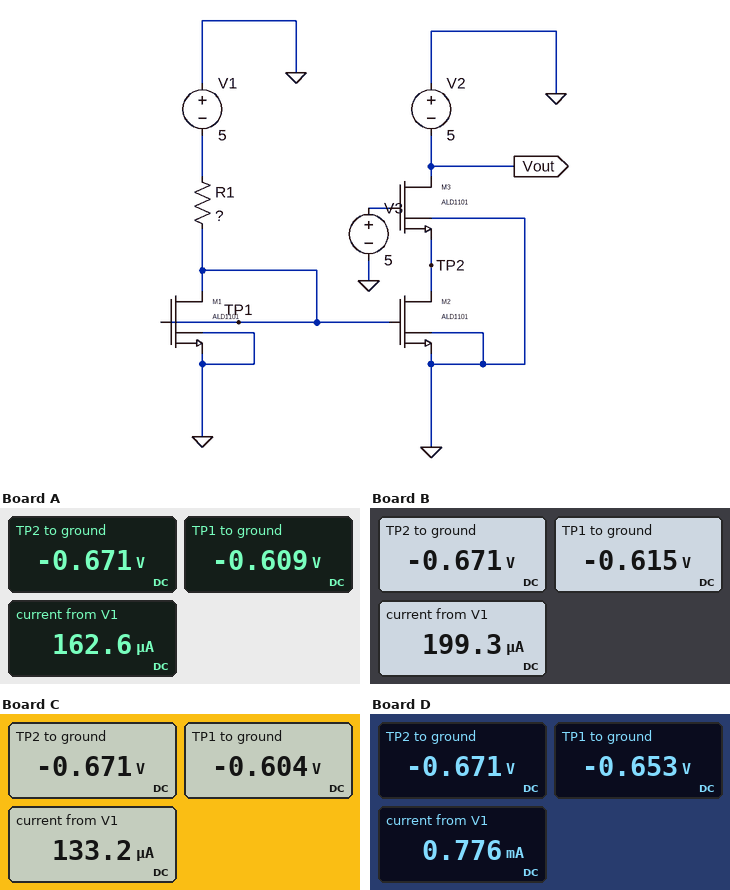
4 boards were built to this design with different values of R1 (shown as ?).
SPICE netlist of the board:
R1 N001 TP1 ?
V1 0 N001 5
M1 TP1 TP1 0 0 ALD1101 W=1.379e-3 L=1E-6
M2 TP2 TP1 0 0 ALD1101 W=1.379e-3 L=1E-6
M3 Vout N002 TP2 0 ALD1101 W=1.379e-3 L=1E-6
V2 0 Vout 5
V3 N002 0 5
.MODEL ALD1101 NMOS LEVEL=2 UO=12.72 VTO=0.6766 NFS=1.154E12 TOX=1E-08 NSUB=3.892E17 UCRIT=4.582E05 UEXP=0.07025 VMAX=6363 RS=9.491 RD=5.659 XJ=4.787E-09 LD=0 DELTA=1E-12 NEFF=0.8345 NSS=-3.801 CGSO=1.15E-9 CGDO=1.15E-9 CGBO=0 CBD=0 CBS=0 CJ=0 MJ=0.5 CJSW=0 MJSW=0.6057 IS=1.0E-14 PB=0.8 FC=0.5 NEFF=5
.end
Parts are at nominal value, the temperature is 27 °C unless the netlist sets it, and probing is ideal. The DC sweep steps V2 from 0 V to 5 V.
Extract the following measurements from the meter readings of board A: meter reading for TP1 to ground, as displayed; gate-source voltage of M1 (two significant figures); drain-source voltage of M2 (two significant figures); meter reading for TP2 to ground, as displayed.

-0.609 V
-610 mV
-670 mV
-0.671 V
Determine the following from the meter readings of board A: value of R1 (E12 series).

27 kΩ
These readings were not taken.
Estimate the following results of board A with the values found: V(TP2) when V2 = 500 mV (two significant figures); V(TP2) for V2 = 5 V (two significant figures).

-500 mV
-670 mV
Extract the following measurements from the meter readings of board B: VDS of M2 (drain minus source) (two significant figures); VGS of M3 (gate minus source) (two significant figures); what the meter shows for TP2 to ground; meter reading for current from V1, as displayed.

-670 mV
5.7 V
-0.671 V
199.3 µA
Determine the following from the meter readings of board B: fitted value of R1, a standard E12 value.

22 kΩ
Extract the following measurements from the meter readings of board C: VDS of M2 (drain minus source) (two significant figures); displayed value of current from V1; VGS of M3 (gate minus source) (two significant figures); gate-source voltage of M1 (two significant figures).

-670 mV
133.2 µA
5.7 V
-600 mV
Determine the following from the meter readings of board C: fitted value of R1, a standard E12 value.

33 kΩ
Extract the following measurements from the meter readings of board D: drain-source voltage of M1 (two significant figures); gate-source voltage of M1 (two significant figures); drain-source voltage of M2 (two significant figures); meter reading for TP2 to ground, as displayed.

-650 mV
-650 mV
-670 mV
-0.671 V
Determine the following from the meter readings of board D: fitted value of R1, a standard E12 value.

5.6 kΩ
